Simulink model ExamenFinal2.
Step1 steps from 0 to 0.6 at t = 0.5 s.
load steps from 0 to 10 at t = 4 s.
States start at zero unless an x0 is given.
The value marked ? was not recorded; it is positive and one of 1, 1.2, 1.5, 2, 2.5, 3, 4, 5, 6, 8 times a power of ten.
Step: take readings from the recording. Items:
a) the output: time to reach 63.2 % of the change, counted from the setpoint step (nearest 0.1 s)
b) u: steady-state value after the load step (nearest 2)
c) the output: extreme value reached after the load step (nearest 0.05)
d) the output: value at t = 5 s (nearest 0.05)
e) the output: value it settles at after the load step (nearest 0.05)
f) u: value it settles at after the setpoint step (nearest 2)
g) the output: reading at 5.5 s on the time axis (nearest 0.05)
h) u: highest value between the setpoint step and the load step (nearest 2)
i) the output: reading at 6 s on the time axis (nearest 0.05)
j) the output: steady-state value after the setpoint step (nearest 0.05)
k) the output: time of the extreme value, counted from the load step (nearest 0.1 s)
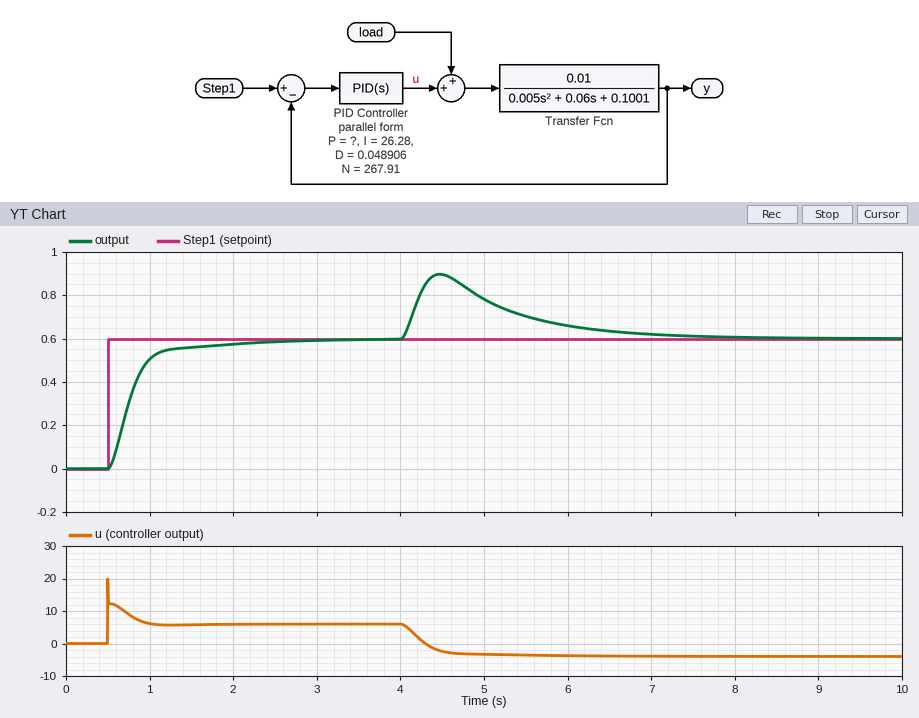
0.3 s
-4
0.90
0.80
0.60
6
0.70
20
0.65
0.60
0.5 s
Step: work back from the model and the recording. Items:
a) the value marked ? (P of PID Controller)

20
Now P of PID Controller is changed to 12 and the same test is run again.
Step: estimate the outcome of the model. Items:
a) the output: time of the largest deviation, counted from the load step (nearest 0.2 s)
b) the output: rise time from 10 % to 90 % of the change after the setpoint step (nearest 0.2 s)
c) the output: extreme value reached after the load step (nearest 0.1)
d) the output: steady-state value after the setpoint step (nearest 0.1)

0.6 s
0.6 s
1.0
0.6
